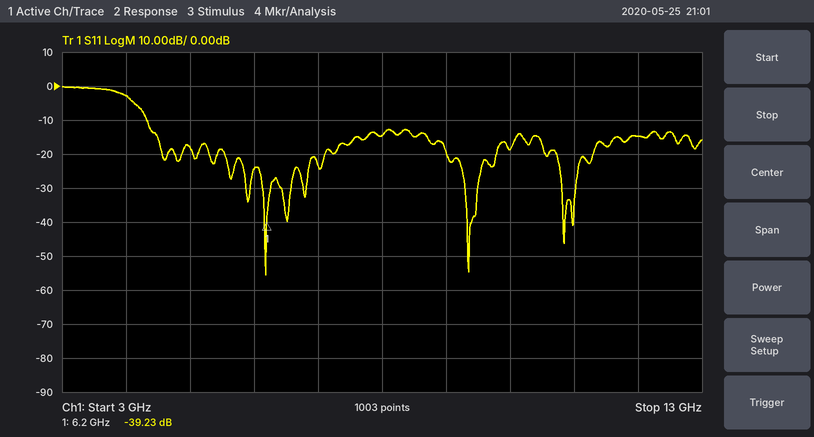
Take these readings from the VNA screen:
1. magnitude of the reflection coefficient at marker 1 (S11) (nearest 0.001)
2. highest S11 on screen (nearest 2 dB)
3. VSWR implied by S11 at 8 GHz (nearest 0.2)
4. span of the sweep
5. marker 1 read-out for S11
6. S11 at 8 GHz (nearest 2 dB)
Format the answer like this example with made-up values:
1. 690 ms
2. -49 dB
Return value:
1. 0.011
2. 0 dB
3. 1.4
4. 10 GHz
5. -39.23 dB
6. -14 dB
